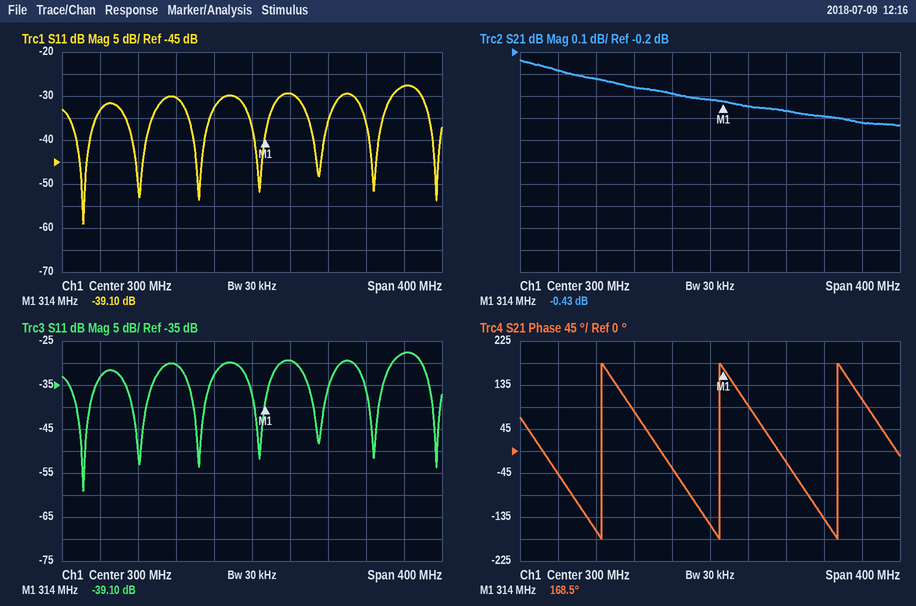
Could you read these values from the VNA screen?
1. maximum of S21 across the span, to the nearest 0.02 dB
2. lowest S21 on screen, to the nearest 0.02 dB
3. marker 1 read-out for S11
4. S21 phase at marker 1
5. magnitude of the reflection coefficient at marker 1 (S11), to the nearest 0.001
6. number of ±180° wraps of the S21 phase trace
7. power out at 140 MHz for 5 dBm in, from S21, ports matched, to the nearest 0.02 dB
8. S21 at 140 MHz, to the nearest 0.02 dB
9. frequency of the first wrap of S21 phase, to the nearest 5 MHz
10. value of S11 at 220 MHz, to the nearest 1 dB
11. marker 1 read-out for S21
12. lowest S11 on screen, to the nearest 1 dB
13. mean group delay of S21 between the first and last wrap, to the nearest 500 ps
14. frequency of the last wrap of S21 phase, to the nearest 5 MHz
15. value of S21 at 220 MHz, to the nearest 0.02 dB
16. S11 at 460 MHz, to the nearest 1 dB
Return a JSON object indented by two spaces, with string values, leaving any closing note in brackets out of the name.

{
  "maximum of S21 across the span, to the nearest 0.02 dB": "-0.24 dB",
  "lowest S21 on screen, to the nearest 0.02 dB": "-0.54 dB",
  "marker 1 read-out for S11": "-39.10 dB",
  "S21 phase at marker 1": "168.5°",
  "magnitude of the reflection coefficient at marker 1 (S11), to the nearest 0.001": "0.011",
  "number of ±180° wraps of the S21 phase trace": "3",
  "power out at 140 MHz for 5 dBm in, from S21, ports matched, to the nearest 0.02 dB": "4.72 dBm",
  "S21 at 140 MHz, to the nearest 0.02 dB": "-0.28 dB",
  "frequency of the first wrap of S21 phase, to the nearest 5 MHz": "185 MHz",
  "value of S11 at 220 MHz, to the nearest 1 dB": "-30 dB",
  "marker 1 read-out for S21": "-0.43 dB",
  "lowest S11 on screen, to the nearest 1 dB": "-59 dB",
  "mean group delay of S21 between the first and last wrap, to the nearest 500 ps": "8.0 ns",
  "frequency of the last wrap of S21 phase, to the nearest 5 MHz": "435 MHz",
  "value of S21 at 220 MHz, to the nearest 0.02 dB": "-0.36 dB",
  "S11 at 460 MHz, to the nearest 1 dB": "-28 dB"
}
